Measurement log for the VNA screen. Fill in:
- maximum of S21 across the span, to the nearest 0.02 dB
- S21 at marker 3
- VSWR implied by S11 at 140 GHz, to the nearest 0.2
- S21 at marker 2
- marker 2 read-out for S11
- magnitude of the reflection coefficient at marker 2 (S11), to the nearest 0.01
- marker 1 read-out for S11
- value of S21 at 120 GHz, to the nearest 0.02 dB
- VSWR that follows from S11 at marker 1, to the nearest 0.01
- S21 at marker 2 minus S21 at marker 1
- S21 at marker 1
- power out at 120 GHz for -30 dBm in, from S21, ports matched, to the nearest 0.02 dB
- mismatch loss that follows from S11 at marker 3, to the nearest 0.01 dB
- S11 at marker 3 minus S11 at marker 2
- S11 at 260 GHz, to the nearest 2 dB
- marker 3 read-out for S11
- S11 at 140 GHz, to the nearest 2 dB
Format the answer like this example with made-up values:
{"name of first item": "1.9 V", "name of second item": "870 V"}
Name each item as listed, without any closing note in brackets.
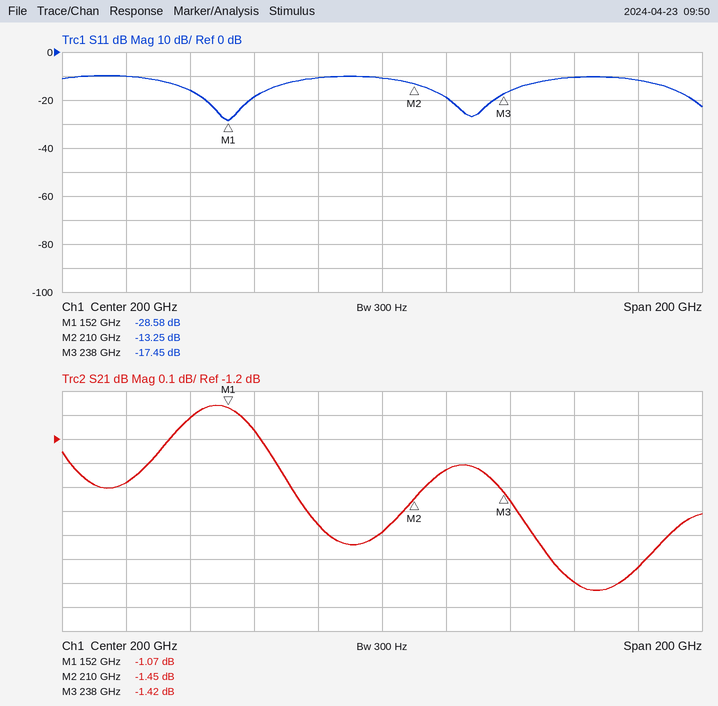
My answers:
{"maximum of S21 across the span, to the nearest 0.02 dB": "-1.06 dB", "S21 at marker 3": "-1.42 dB", "VSWR implied by S11 at 140 GHz, to the nearest 0.2": "1.4", "S21 at marker 2": "-1.45 dB", "marker 2 read-out for S11": "-13.25 dB", "magnitude of the reflection coefficient at marker 2 (S11), to the nearest 0.01": "0.22", "marker 1 read-out for S11": "-28.58 dB", "value of S21 at 120 GHz, to the nearest 0.02 dB": "-1.38 dB", "VSWR that follows from S11 at marker 1, to the nearest 0.01": "1.08", "S21 at marker 2 minus S21 at marker 1": "-0.38 dB", "S21 at marker 1": "-1.07 dB", "power out at 120 GHz for -30 dBm in, from S21, ports matched, to the nearest 0.02 dB": "-31.38 dBm", "mismatch loss that follows from S11 at marker 3, to the nearest 0.01 dB": "0.08 dB", "S11 at marker 3 minus S11 at marker 2": "-4.20 dB", "S11 at 260 GHz, to the nearest 2 dB": "-10 dB", "marker 3 read-out for S11": "-17.45 dB", "S11 at 140 GHz, to the nearest 2 dB": "-16 dB"}
